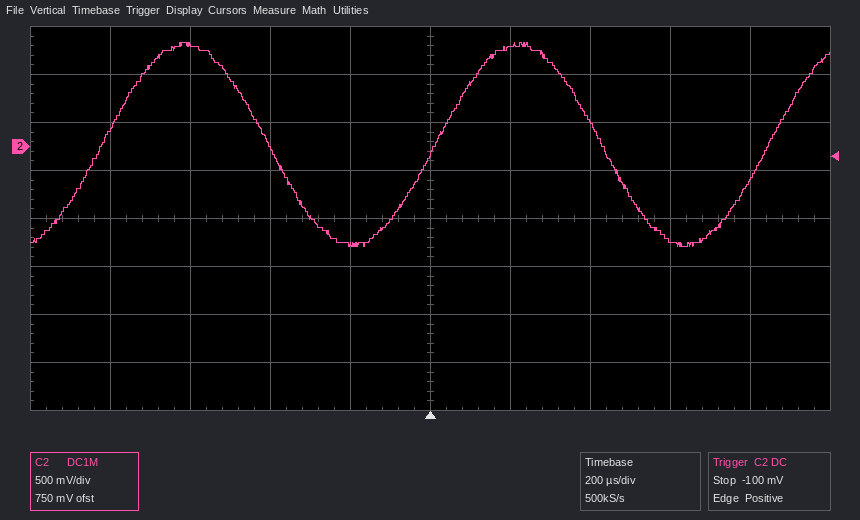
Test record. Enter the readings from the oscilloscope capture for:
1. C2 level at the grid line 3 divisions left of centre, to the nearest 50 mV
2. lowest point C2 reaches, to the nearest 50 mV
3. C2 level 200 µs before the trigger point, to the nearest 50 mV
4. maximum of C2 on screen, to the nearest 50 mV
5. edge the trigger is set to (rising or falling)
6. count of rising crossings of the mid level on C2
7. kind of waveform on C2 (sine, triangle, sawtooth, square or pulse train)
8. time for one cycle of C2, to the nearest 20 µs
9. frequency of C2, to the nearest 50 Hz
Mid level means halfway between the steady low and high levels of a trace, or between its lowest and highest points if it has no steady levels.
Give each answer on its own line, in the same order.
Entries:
1.05 V
-1.05 V
-1.00 V
1.10 V
rising
3
sine
840 µs
1.20 kHz
